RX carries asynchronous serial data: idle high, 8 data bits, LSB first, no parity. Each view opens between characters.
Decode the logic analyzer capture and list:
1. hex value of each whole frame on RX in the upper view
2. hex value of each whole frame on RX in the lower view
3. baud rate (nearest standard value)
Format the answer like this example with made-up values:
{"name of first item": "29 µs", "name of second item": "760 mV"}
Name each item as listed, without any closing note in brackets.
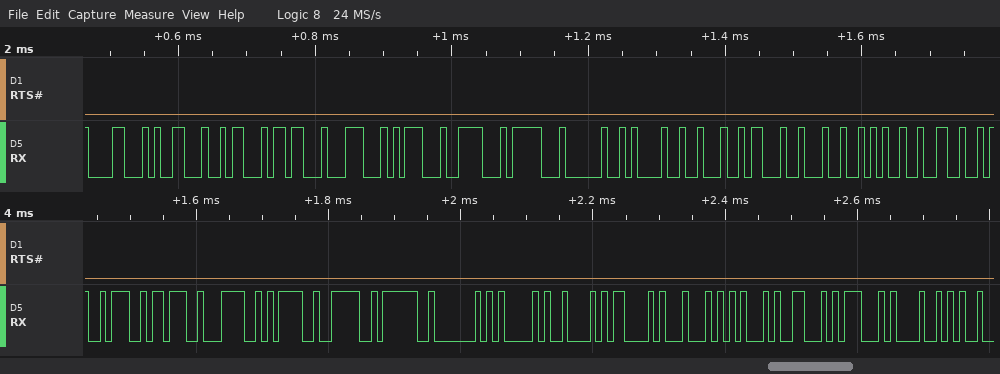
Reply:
{"hex value of each whole frame on RX in the upper view": "18, 19, 1A, 1B, 1C, 1D, 1E, 1F, 20, 21, 22, 23, 24, 25, 26", "hex value of each whole frame on RX in the lower view": "3A, 3B, 3C, 3D, 3E, 3F, 40, 41, 42, 43, 44, 45, 46, 47, 48", "baud rate": "115200 baud"}
